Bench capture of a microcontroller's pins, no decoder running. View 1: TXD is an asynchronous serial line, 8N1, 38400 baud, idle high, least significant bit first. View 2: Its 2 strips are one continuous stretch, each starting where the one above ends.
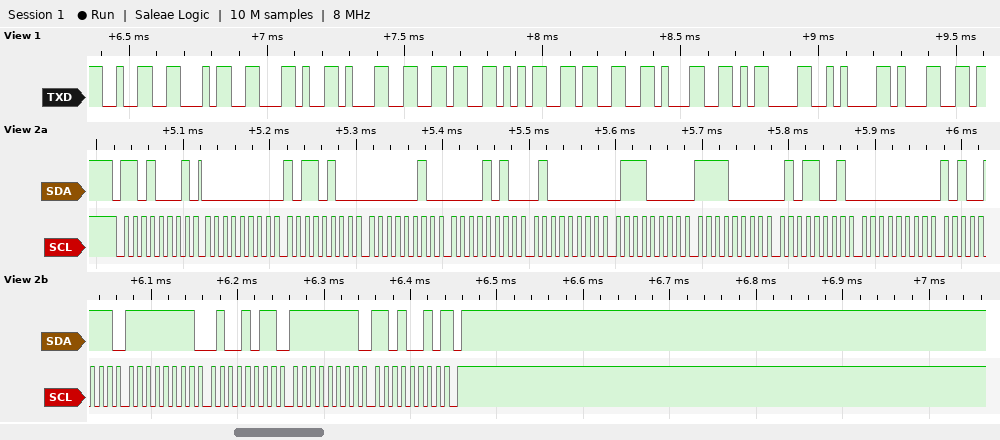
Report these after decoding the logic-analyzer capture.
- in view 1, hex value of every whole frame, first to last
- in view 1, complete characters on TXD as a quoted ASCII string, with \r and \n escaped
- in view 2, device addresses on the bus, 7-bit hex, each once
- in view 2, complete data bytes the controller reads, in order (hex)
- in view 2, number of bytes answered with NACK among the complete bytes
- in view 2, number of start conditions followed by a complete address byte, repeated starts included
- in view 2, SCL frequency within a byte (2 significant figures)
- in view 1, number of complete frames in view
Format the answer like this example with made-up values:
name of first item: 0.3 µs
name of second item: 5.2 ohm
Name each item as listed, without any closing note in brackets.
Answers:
in view 1, hex value of every whole frame, first to last: 0x32 0x34 0x2C 0x31 0x36 0x35 0x33 0x31 0x0D 0x0A 0x31
in view 1, complete characters on TXD as a quoted ASCII string, with \r and \n escaped: "24,16531\r\n1"
in view 2, device addresses on the bus, 7-bit hex, each once: 0x68
in view 2, complete data bytes the controller reads, in order: 00 B4 02 0A 40 70 F0 59 00 A7 FF 4B FF D2
in view 2, number of bytes answered with NACK among the complete bytes: 1
in view 2, number of start conditions followed by a complete address byte, repeated starts included: 1
in view 2, SCL frequency within a byte: 100 kHz
in view 1, number of complete frames in view: 11
